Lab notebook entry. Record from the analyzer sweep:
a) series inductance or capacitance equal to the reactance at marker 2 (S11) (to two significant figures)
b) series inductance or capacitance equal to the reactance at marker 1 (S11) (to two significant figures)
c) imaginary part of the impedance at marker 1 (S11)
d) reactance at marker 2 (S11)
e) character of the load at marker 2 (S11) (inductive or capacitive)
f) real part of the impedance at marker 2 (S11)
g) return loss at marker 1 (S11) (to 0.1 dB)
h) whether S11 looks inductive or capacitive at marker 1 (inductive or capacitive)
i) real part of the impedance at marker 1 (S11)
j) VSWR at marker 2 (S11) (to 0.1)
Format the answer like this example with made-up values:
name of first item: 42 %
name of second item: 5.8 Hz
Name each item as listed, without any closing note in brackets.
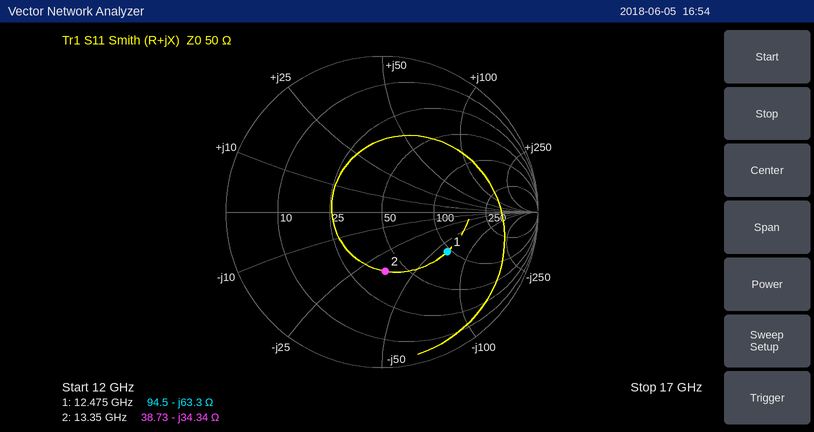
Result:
series inductance or capacitance equal to the reactance at marker 2 (S11): 350 fF
series inductance or capacitance equal to the reactance at marker 1 (S11): 200 fF
imaginary part of the impedance at marker 1: -63.3 Ω
reactance at marker 2: -34.34 Ω
character of the load at marker 2 (S11): capacitive
real part of the impedance at marker 2: 38.73 Ω
return loss at marker 1 (S11): 6.2 dB
whether S11 looks inductive or capacitive at marker 1: capacitive
real part of the impedance at marker 1: 94.5 Ω
VSWR at marker 2 (S11): 2.2
